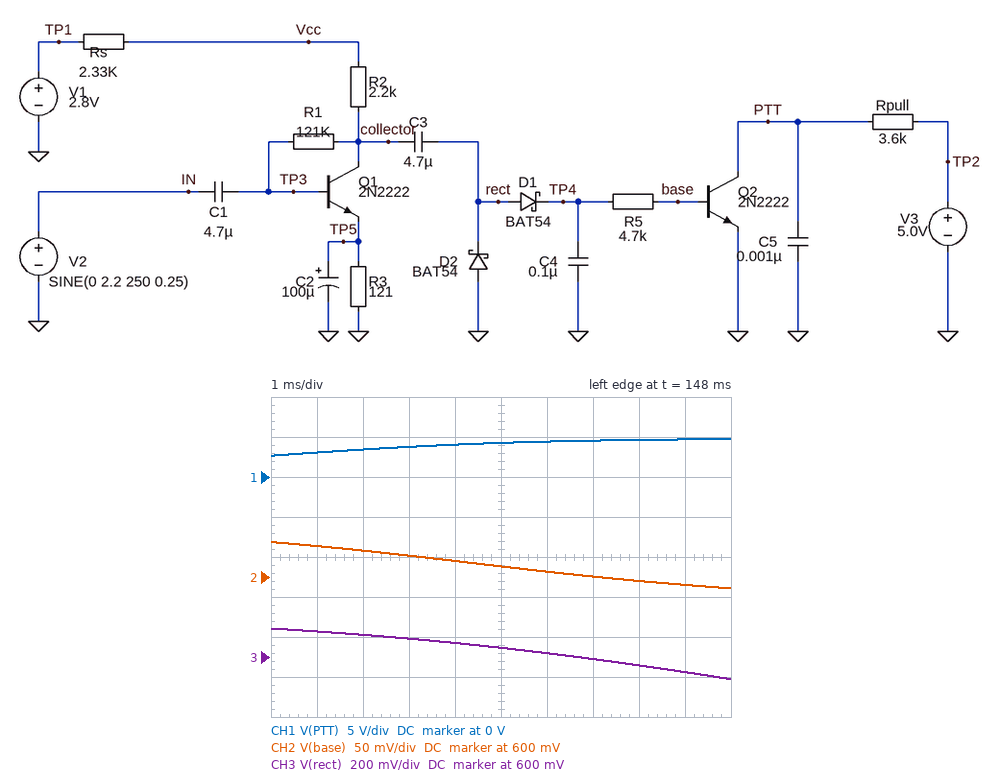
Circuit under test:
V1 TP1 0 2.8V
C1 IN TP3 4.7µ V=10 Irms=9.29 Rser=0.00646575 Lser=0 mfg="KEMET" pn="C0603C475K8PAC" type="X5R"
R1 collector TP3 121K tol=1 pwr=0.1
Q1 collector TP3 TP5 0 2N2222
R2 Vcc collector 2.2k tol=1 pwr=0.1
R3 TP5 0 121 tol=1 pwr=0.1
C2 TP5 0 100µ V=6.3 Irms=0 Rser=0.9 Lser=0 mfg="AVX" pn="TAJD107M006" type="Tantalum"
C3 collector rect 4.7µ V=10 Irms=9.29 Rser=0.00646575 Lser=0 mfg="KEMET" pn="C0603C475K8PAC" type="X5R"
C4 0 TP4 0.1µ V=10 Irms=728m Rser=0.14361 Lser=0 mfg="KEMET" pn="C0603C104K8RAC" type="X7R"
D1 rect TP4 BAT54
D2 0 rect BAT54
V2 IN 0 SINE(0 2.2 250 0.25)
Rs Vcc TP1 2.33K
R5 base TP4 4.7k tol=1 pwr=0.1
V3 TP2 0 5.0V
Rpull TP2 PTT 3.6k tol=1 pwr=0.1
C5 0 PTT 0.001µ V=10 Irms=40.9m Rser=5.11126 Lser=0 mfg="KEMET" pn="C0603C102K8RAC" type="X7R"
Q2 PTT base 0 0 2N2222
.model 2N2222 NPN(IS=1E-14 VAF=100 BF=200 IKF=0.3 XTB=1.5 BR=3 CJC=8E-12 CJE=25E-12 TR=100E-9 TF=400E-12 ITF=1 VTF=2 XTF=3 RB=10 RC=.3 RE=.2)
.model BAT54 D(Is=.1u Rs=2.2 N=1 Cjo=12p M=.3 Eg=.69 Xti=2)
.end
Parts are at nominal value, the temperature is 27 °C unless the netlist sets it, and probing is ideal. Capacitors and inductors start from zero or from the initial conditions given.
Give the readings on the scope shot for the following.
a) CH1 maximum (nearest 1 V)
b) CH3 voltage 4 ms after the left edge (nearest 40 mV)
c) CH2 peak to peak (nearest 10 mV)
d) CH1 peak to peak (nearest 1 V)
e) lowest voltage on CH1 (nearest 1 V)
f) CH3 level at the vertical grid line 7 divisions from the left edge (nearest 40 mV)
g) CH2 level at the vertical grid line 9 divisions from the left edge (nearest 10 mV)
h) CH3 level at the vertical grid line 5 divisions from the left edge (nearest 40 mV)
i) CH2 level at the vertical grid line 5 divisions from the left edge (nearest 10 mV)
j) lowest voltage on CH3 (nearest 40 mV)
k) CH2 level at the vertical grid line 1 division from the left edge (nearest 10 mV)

5 V
680 mV
60 mV
2 V
3 V
600 mV
590 mV
640 mV
610 mV
480 mV
640 mV
